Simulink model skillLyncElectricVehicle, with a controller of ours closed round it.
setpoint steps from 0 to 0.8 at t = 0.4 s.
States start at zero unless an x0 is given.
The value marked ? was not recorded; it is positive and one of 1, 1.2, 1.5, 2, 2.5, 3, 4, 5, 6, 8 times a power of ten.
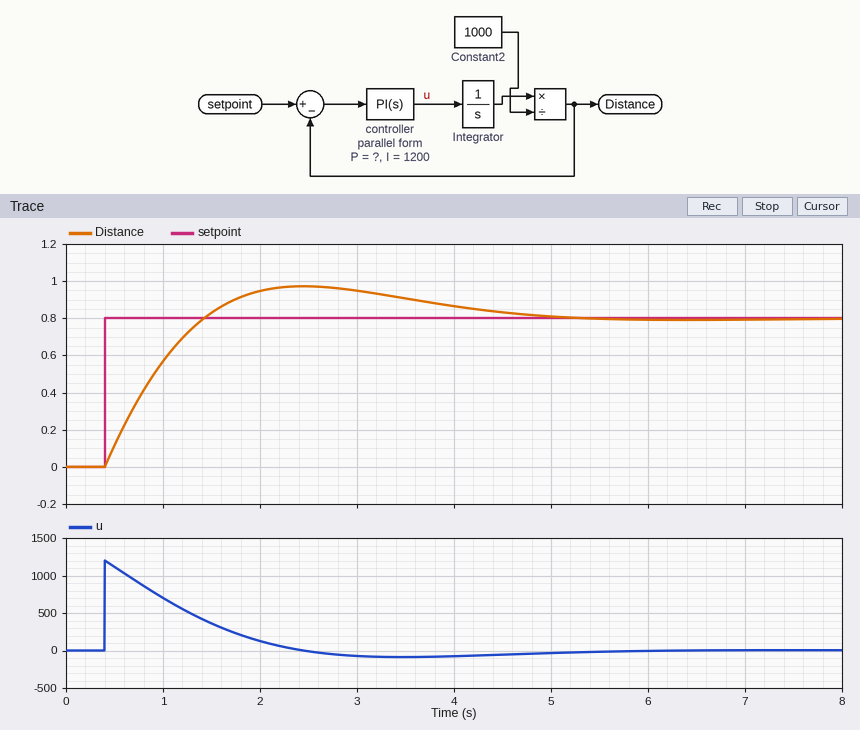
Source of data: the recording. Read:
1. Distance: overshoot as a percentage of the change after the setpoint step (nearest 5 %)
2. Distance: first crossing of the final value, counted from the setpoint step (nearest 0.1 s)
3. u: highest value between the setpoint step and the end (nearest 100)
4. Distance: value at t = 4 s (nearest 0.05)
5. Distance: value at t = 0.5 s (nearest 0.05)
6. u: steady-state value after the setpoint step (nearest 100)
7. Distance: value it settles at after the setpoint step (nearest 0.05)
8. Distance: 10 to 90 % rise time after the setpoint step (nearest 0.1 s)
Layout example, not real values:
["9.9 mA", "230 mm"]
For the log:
["20 %", "1.0 s", "1200", "0.85", "0.10", "0", "0.80", "0.8 s"]
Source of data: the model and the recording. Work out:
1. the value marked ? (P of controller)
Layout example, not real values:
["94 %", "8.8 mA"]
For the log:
["1500"]
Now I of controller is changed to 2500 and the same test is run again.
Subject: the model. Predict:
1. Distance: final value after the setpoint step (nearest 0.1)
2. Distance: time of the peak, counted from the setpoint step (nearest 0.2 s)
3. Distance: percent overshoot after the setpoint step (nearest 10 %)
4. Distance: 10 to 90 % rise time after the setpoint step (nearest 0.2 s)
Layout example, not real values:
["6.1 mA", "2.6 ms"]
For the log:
["0.8", "1.6 s", "30 %", "0.6 s"]
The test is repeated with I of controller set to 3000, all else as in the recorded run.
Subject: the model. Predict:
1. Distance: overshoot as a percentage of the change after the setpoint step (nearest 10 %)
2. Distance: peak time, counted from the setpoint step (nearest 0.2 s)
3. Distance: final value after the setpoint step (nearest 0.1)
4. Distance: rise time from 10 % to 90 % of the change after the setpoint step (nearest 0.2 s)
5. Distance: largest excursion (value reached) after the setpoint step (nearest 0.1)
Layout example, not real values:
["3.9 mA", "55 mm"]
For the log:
["30 %", "1.4 s", "0.8", "0.6 s", "1.1"]
